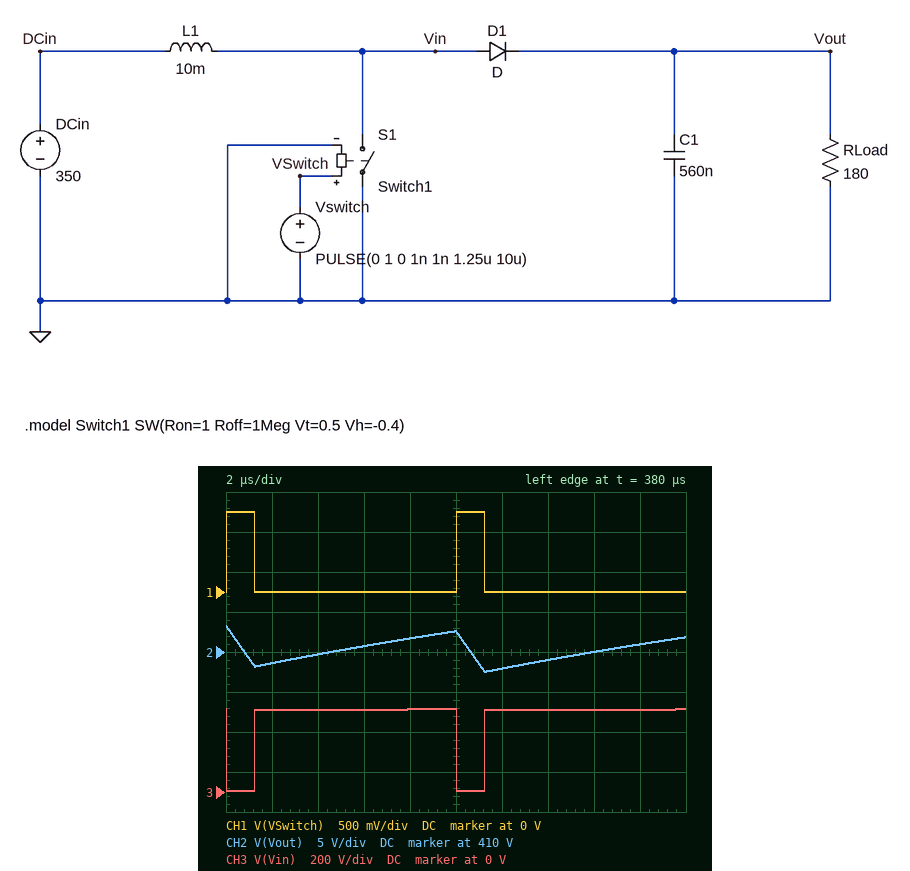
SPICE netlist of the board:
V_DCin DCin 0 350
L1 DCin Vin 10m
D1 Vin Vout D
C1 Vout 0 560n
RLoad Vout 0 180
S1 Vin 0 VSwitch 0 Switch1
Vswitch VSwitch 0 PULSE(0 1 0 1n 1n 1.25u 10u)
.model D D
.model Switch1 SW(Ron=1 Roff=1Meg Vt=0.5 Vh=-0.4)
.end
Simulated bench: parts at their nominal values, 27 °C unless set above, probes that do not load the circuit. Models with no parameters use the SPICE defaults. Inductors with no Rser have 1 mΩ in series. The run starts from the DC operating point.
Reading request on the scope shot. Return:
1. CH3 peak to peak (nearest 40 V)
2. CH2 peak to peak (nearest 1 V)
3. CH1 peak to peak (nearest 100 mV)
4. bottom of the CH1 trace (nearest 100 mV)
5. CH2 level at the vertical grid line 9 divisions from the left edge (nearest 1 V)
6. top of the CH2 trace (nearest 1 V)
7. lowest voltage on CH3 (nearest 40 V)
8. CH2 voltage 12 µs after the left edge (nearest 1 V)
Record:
400 V
6 V
1.0 V
0 V
411 V
413 V
0 V
408 V
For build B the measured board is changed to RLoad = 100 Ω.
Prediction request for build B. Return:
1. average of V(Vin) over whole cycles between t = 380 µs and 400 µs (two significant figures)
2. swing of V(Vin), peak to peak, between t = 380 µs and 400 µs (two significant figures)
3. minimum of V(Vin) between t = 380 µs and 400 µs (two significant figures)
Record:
350 V
400 V
4.6 V
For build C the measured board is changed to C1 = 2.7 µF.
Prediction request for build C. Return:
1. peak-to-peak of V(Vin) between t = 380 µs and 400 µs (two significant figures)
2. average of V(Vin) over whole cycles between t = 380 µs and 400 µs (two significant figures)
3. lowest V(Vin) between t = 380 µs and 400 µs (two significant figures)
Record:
400 V
350 V
3.1 V
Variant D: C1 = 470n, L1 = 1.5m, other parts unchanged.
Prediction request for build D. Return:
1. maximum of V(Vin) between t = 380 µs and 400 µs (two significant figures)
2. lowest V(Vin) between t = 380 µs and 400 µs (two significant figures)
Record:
400 V
2.3 V
